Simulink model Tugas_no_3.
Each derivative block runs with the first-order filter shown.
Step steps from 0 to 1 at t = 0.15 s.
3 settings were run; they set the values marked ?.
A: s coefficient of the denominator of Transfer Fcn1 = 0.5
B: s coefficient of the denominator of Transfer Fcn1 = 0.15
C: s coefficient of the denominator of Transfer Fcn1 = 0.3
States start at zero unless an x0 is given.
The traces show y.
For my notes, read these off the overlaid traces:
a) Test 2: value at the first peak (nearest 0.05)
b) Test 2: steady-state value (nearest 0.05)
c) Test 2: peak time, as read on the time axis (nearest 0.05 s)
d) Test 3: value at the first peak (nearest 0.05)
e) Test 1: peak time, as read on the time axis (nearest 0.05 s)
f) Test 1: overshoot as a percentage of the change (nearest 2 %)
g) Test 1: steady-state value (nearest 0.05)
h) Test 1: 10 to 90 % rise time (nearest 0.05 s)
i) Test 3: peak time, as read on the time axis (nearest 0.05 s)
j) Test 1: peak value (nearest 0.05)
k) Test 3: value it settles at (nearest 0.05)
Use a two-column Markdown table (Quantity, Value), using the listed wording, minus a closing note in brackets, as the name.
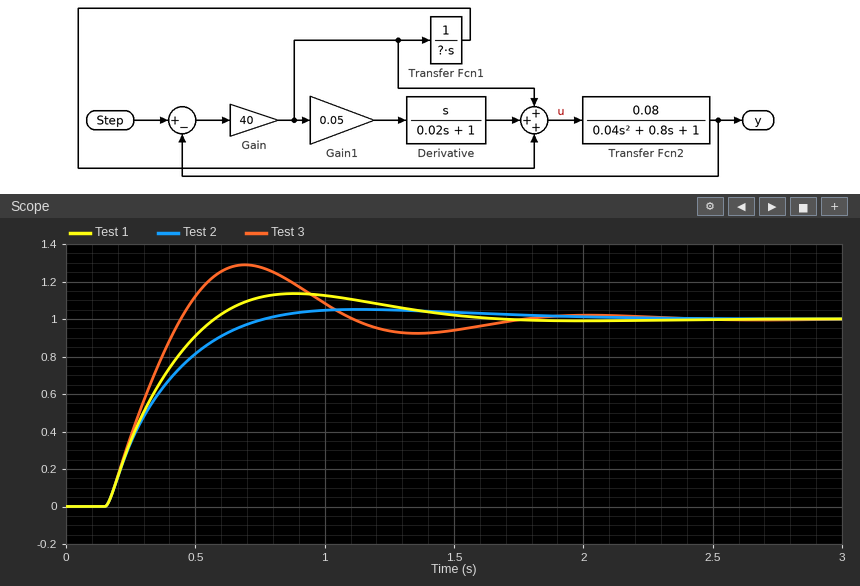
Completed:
| Quantity | Value |
|---|---|
| Test 2: value at the first peak | 1.05 |
| Test 2: steady-state value | 1.00 |
| Test 2: peak time, as read on the time axis | 1.15 s |
| Test 3: value at the first peak | 1.30 |
| Test 1: peak time, as read on the time axis | 0.90 s |
| Test 1: overshoot as a percentage of the change | 14 % |
| Test 1: steady-state value | 1.00 |
| Test 1: 10 to 90 % rise time | 0.30 s |
| Test 3: peak time, as read on the time axis | 0.70 s |
| Test 1: peak value | 1.15 |
| Test 3: value it settles at | 1.00 |
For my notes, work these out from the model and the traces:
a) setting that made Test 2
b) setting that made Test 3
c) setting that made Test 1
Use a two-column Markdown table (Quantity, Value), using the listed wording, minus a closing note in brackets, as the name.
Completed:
| Quantity | Value |
|---|---|
| setting that made Test 2 | A |
| setting that made Test 3 | B |
| setting that made Test 1 | C |
